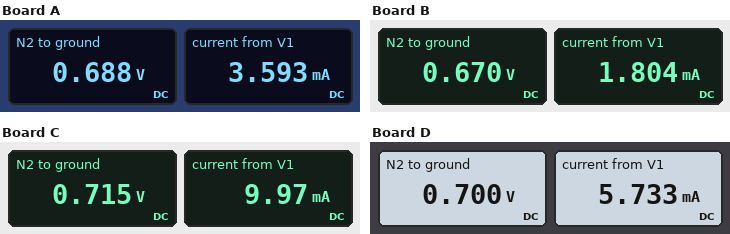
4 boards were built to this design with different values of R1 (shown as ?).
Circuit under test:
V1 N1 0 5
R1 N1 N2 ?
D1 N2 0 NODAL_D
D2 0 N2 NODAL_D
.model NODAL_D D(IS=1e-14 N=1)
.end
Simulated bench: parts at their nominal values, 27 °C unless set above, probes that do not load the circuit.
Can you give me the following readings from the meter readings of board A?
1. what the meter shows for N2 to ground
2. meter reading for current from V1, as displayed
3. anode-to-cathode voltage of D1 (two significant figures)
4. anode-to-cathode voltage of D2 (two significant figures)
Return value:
0.688 V
3.593 mA
690 mV
-690 mV
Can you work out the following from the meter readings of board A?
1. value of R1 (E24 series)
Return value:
1.2 kΩ
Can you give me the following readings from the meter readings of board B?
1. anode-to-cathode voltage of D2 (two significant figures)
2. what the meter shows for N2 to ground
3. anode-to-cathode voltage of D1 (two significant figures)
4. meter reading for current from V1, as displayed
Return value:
-670 mV
0.670 V
670 mV
1.804 mA
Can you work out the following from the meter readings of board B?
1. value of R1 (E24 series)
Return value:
2.4 kΩ
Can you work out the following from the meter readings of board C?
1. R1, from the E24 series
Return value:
430 Ω
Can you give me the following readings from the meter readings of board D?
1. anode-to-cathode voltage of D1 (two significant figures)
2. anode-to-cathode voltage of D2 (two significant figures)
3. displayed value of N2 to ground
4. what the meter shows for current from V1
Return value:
700 mV
-700 mV
0.700 V
5.733 mA
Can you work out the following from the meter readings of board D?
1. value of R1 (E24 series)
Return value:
750 Ω
